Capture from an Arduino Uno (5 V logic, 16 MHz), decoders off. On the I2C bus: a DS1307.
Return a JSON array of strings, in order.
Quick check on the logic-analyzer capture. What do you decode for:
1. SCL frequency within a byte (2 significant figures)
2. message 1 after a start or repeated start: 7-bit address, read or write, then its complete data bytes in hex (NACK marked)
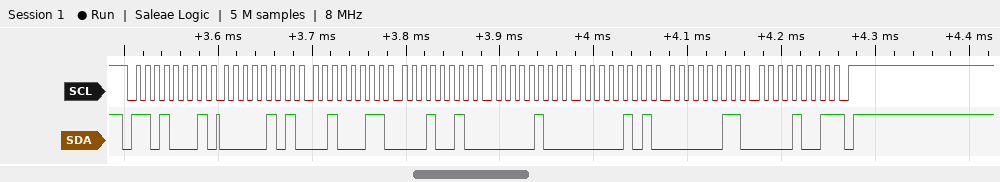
["100 kHz", "0x68 read: 05 23 12 04 05 03 09 NACK"]
